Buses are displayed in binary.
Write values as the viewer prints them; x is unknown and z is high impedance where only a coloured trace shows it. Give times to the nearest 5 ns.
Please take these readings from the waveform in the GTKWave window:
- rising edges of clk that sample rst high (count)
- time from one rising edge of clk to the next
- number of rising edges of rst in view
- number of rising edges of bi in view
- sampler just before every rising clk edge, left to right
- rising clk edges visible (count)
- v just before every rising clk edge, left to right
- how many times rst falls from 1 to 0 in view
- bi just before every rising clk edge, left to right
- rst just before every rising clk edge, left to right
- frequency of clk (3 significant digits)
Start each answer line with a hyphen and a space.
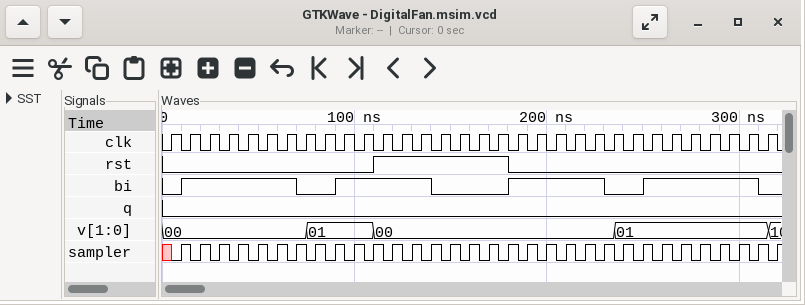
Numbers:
- 7
- 10 ns
- 1
- 4
- x 1 1 1 1 1 1 1 1 1 1 1 1 1 1 1 1 1 1 1 1 1 1 1 1 1 1 1 1 1 1 1
- 32
- 00, 00, 00, 00, 00, 00, 00, 00, 01, 01, 01, 00, 00, 00, 00, 00, 00, 00, 00, 00, 00, 00, 00, 00, 01, 01, 01, 01, 01, 01, 01, 01
- 1
- 0 1 1 1 1 1 1 0 0 1 1 1 1 1 0 0 0 0 1 1 1 1 1 0 0 1 1 1 1 1 1 0
- 0 0 0 0 0 0 0 0 0 0 0 1 1 1 1 1 1 1 0 0 0 0 0 0 0 0 0 0 0 0 0 0
- 100 MHz
